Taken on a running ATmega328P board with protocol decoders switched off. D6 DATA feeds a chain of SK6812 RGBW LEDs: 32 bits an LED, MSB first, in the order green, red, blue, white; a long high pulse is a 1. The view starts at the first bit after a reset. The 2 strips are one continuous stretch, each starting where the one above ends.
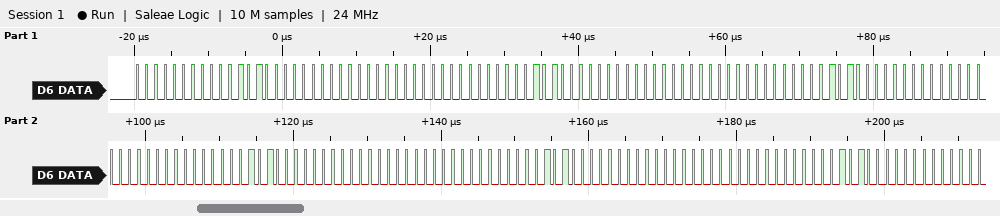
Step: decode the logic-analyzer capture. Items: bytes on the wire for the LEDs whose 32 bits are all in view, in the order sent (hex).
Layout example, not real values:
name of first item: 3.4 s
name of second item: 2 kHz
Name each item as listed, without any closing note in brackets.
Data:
bytes on the wire for the LEDs whose 32 bits are all in view, in the order sent: 00 14 00 00 00 14 00 00 00 14 00 00 00 14 00 00 00 14 00 00
